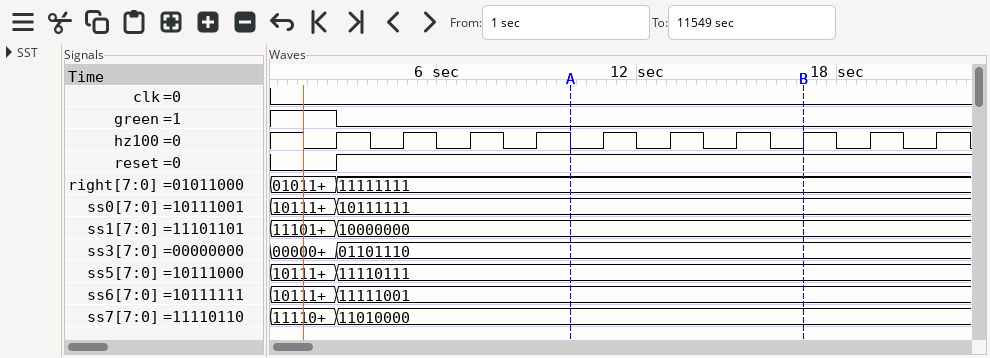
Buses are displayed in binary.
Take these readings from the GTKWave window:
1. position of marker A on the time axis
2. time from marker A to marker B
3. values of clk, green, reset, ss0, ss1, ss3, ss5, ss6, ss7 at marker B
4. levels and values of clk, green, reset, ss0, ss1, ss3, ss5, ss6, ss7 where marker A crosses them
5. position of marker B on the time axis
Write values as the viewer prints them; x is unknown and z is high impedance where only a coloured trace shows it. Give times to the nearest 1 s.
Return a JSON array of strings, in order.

["10 s", "7 s", "clk=0, green=0, reset=1, ss0=10111111, ss1=10000000, ss3=01101110, ss5=11110111, ss6=11111001, ss7=11010000", "clk=0, green=0, reset=1, ss0=10111111, ss1=10000000, ss3=01101110, ss5=11110111, ss6=11111001, ss7=11010000", "17 s"]
